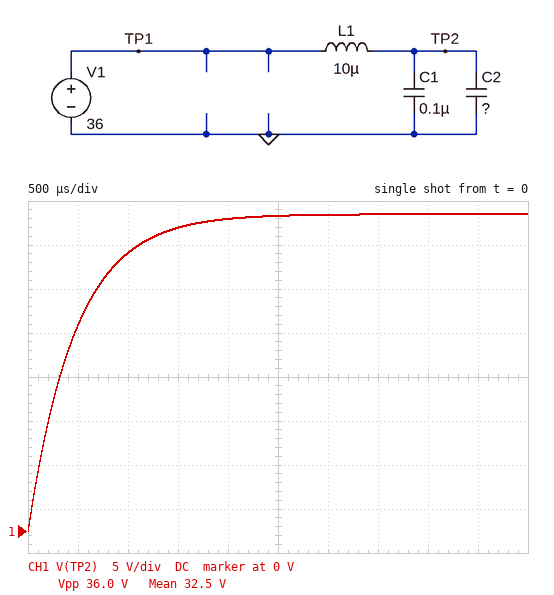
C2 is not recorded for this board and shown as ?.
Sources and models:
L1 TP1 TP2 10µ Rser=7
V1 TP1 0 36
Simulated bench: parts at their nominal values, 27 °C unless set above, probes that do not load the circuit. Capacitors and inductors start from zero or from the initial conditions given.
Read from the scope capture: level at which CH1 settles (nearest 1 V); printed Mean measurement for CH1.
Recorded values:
36 V
32.5 V
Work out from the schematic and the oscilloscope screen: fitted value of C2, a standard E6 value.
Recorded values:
68 µF
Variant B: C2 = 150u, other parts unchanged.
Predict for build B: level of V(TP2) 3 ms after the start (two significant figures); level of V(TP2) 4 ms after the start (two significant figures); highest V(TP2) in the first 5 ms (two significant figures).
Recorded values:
34 V
35 V
36 V
